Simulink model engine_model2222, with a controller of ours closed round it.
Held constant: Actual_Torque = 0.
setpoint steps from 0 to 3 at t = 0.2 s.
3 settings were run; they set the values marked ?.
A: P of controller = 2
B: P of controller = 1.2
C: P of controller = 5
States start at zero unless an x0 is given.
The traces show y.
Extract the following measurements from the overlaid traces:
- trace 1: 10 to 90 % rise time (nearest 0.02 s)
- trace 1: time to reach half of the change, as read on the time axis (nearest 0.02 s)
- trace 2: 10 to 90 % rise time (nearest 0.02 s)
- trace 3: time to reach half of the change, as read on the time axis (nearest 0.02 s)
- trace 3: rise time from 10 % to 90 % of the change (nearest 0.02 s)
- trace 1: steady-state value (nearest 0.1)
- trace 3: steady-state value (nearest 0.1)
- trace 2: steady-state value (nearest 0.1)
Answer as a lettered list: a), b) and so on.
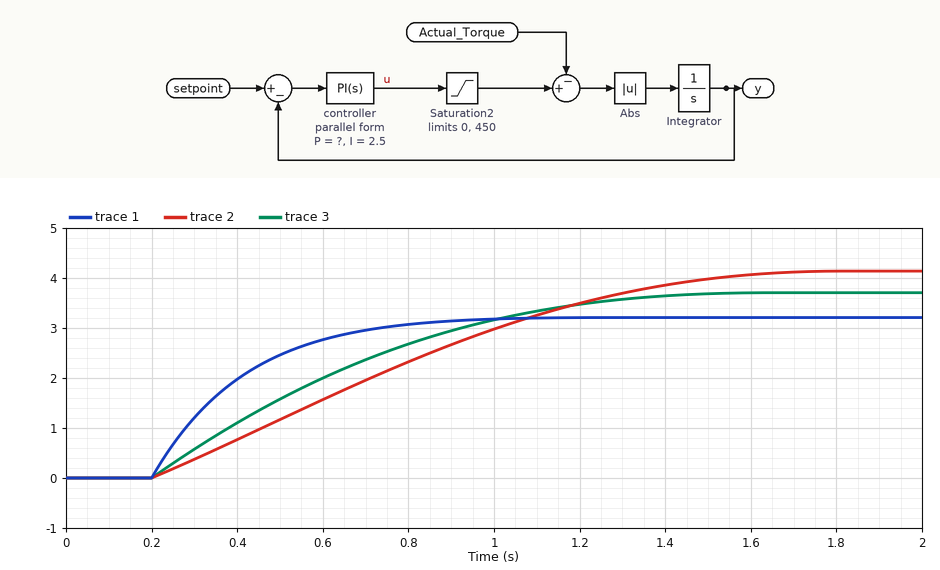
a) 0.44 s
b) 0.34 s
c) 1.00 s
d) 0.56 s
e) 0.84 s
f) 3.2
g) 3.7
h) 4.1
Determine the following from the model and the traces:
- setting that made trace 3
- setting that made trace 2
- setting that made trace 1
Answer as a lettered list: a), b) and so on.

a) A
b) B
c) C
